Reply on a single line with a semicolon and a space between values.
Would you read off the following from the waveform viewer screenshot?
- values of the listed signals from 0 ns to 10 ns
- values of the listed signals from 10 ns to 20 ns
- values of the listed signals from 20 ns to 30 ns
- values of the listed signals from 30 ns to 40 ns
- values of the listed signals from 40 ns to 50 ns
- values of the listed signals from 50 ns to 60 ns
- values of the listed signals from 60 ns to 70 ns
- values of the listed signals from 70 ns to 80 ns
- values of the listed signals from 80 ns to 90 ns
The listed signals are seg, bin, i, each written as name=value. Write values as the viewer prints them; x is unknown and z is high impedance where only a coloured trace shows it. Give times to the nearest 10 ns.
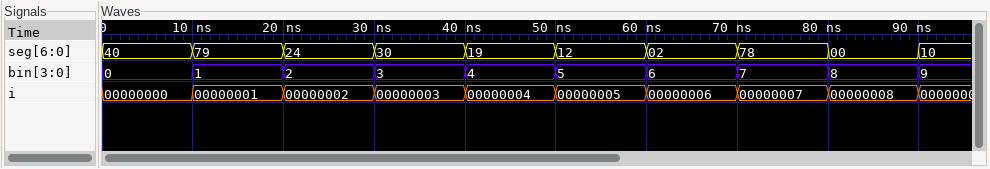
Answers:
seg=40, bin=0, i=00000000; seg=79, bin=1, i=00000001; seg=24, bin=2, i=00000002; seg=30, bin=3, i=00000003; seg=19, bin=4, i=00000004; seg=12, bin=5, i=00000005; seg=02, bin=6, i=00000006; seg=78, bin=7, i=00000007; seg=00, bin=8, i=00000008
